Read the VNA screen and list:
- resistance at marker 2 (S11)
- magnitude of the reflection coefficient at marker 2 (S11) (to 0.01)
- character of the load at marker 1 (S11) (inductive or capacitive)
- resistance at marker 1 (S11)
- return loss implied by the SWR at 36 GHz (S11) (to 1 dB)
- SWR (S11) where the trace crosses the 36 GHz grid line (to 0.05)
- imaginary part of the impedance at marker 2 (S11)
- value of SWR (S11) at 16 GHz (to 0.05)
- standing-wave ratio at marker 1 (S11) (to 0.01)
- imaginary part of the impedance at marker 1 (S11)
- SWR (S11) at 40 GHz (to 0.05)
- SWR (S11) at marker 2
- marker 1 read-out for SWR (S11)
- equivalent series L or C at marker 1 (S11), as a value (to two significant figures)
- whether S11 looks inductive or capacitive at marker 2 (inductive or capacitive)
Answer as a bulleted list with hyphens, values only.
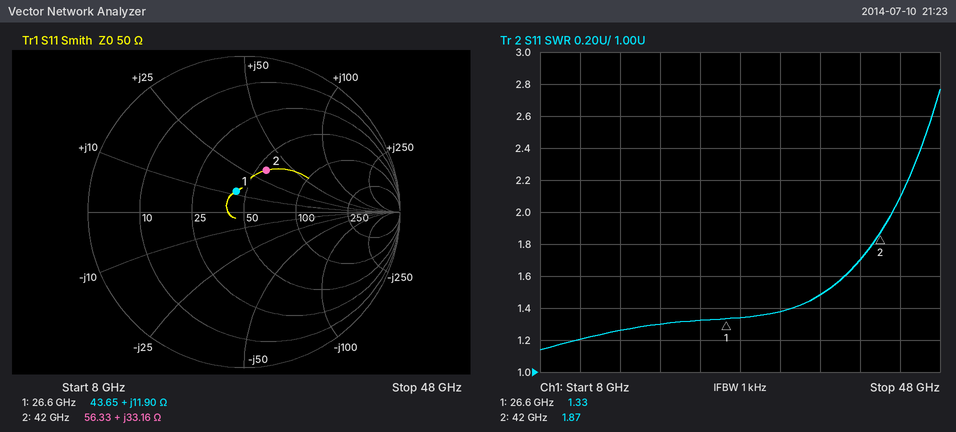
- 56.33 Ω
- 0.30
- inductive
- 43.65 Ω
- 14 dB
- 1.50
- +33.16 Ω
- 1.25
- 1.33
- +11.90 Ω
- 1.70
- 1.87
- 1.33
- 71 pH
- inductive
